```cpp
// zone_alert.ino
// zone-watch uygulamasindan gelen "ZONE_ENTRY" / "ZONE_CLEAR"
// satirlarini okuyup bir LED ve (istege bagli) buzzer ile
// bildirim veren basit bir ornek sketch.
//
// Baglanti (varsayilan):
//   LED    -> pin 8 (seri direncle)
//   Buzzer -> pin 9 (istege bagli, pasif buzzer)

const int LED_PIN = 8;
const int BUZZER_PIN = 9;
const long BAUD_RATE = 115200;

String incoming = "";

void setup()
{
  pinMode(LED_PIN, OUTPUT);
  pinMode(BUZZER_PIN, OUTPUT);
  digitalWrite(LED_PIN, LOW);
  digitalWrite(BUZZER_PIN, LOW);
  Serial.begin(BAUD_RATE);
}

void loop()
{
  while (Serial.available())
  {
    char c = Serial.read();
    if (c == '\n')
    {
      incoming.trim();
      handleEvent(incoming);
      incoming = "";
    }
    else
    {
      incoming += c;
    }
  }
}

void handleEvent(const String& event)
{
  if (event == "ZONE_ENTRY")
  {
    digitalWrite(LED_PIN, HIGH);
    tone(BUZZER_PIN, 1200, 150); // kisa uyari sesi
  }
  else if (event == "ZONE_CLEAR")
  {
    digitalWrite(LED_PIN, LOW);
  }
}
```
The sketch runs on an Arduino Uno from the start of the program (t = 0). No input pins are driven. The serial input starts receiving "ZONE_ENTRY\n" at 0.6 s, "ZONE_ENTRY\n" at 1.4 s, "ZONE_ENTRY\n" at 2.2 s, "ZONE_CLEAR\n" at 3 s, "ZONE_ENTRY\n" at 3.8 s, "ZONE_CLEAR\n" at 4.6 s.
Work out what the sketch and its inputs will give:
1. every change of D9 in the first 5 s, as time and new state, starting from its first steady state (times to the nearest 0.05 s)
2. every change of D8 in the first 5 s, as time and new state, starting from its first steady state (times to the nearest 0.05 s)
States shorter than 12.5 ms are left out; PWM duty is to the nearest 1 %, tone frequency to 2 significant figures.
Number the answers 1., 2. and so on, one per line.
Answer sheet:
1. 0 s low; 0.6 s tone 1200 Hz; 0.75 s low; 1.4 s tone 1200 Hz; 1.55 s low; 2.2 s tone 1200 Hz; 2.35 s low; 3.8 s tone 1200 Hz; 3.95 s low
2. 0 s low; 0.6 s high; 3 s low; 3.8 s high; 4.6 s low
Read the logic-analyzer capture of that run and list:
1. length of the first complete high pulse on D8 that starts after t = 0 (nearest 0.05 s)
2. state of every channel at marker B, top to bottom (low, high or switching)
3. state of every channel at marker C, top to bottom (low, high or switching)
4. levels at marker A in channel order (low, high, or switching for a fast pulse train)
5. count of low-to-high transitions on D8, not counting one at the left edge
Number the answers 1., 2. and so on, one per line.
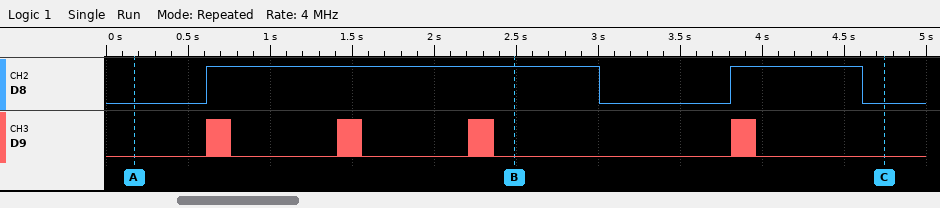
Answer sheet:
1. 2.40 s
2. D8 high, D9 low
3. D8 low, D9 low
4. D8 low, D9 low
5. 2
